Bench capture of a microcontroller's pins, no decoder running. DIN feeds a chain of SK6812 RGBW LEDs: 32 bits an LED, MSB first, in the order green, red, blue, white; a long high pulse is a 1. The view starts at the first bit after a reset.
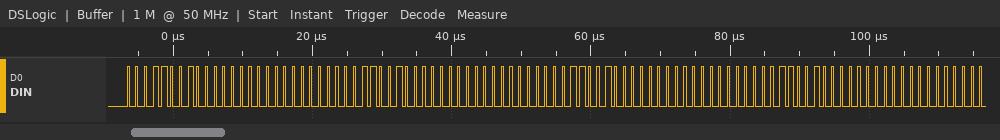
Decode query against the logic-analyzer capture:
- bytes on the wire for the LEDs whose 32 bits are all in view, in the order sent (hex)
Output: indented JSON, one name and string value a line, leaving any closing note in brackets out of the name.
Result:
{
  "bytes on the wire for the LEDs whose 32 bits are all in view, in the order sent": "19 00 00 19 00 00 19 00 00 19 00 00"
}
